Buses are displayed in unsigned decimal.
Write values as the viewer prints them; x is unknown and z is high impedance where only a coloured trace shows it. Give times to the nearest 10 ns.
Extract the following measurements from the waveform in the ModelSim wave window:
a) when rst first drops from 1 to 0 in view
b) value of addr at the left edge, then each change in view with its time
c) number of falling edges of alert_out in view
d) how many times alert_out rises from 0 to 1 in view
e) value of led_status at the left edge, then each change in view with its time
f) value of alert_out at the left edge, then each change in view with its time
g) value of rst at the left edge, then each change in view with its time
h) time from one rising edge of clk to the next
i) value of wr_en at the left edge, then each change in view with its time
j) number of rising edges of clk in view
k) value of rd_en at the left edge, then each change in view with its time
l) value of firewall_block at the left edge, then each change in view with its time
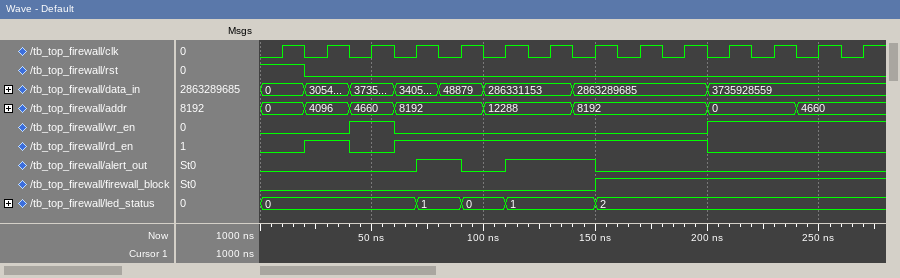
20 ns
0, 4096 at 20 ns, 4660 at 40 ns, 8192 at 60 ns, 12288 at 100 ns, 8192 at 140 ns, 0 at 200 ns, 4660 at 240 ns
2
2
0, 1 at 70 ns, 0 at 90 ns, 1 at 110 ns, 2 at 150 ns
0, 1 at 70 ns, 0 at 90 ns, 1 at 110 ns, 0 at 150 ns
1, 0 at 20 ns
20 ns
0, 1 at 40 ns, 0 at 60 ns, 1 at 200 ns
14
0, 1 at 20 ns, 0 at 40 ns, 1 at 60 ns, 0 at 200 ns
0, 1 at 150 ns
